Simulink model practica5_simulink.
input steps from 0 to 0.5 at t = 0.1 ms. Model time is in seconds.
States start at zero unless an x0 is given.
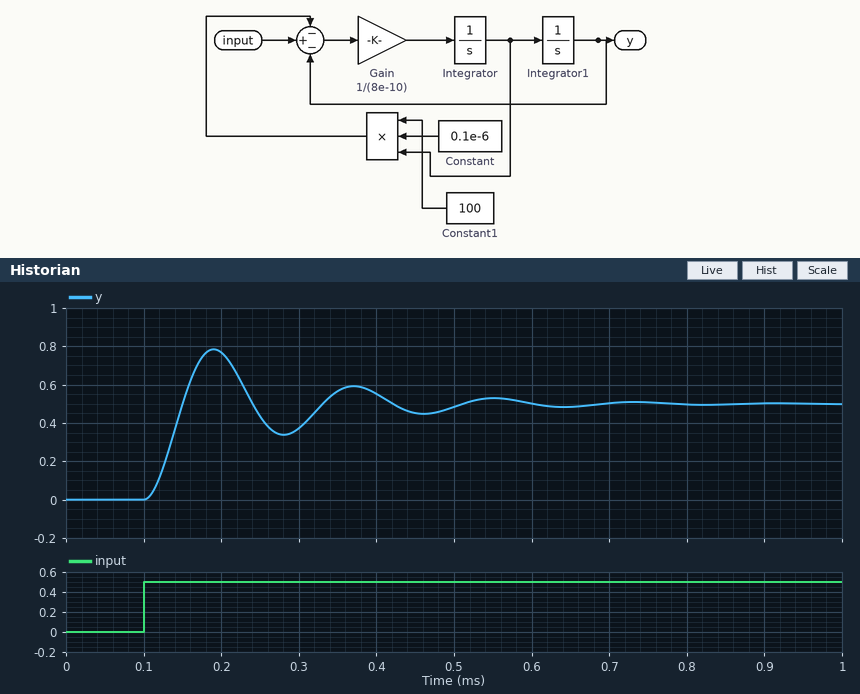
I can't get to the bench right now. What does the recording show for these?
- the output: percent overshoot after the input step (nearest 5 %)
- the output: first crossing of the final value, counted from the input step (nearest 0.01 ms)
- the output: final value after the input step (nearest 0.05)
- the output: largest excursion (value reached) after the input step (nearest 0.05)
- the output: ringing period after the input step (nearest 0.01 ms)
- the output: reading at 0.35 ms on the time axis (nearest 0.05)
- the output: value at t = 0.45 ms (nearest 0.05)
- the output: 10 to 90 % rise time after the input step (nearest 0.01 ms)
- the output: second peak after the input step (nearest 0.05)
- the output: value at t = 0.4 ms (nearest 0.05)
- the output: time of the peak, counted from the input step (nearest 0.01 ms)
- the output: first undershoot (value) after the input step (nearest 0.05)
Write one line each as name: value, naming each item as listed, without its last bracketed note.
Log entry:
the output: percent overshoot after the input step: 55 %
the output: first crossing of the final value, counted from the input step: 0.05 ms
the output: final value after the input step: 0.50
the output: largest excursion (value reached) after the input step: 0.80
the output: ringing period after the input step: 0.18 ms
the output: reading at 0.35 ms on the time axis: 0.55
the output: value at t = 0.45 ms: 0.45
the output: 10 to 90 % rise time after the input step: 0.03 ms
the output: second peak after the input step: 0.60
the output: value at t = 0.4 ms: 0.55
the output: time of the peak, counted from the input step: 0.09 ms
the output: first undershoot (value) after the input step: 0.35
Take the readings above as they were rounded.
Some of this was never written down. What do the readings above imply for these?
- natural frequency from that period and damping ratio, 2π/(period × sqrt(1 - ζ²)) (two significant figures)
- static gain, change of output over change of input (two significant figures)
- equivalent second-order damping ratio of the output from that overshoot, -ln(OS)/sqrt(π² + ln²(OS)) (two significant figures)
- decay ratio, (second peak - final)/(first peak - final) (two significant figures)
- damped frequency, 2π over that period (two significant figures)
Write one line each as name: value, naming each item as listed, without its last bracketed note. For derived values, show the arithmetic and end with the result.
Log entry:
natural frequency from that period and damping ratio, 2π/(period × sqrt(1 - ζ²)): 2π / (0.18 × sqrt(1 - 0.19²)) = 36 rad/ms
static gain, change of output over change of input: (0.5 - 0) / (0.5 - 0) = 1.0
equivalent second-order damping ratio of the output from that overshoot, -ln(OS)/sqrt(π² + ln²(OS)): ln(0.55) = -0.598; 0.598 / sqrt(9.870 + 0.357) = 0.19
decay ratio, (second peak - final)/(first peak - final): (0.6 - 0.5) / (0.8 - 0.5) = 0.33
damped frequency, 2π over that period: 2π / 0.18 = 35 rad/ms
